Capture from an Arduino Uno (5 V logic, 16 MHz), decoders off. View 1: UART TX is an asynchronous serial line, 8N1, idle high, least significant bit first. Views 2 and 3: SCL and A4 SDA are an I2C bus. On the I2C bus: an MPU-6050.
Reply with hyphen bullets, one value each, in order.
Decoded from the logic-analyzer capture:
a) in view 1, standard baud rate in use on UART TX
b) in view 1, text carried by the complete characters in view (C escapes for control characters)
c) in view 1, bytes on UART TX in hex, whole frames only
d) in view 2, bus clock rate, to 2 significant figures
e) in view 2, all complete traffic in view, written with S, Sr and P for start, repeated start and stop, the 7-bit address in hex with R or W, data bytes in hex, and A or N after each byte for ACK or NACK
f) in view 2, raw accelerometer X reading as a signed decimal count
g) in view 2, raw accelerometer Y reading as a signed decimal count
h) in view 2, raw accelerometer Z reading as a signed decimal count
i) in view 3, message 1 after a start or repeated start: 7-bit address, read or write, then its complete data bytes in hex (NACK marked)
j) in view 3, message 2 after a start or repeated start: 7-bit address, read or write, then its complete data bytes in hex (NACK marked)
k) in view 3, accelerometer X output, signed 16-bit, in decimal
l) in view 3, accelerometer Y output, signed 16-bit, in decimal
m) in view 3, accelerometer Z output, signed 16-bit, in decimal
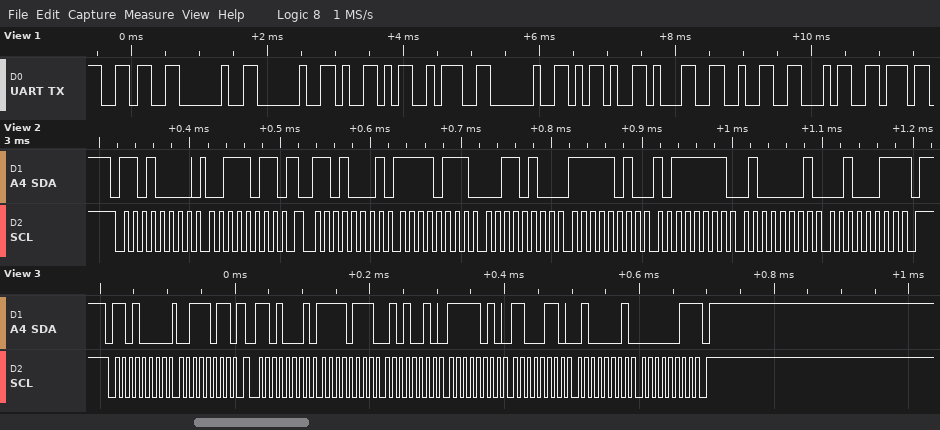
- 9600 baud
- "6  Y: -124"
- 0x36 0x20 0x20 0x59 0x3A 0x20 0x2D 0x31 0x32 0x34
- 100 kHz
- S 68W A 3B A Sr 68R A F7 A 34 A FA A BF A 41 A 23 N P
- -2252
- -1345
- 16675
- 0x68 write: 3B
- 0x68 read: F7 52 FA C6 41 03 NACK
- -2222
- -1338
- 16643
